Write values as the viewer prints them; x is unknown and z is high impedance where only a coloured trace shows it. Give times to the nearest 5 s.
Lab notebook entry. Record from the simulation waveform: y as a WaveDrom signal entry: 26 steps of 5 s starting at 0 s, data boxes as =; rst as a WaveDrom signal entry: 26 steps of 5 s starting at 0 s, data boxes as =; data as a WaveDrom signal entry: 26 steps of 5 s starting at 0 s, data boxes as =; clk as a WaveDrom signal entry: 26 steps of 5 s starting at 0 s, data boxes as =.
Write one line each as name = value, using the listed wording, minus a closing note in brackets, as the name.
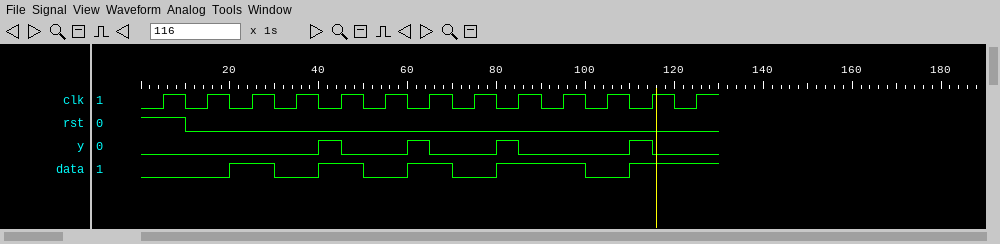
y as a WaveDrom signal entry: 26 steps of 5 s starting at 0 s, data boxes as = = {name: 'y', wave: '0.......10..10..10....10..'}
rst as a WaveDrom signal entry: 26 steps of 5 s starting at 0 s, data boxes as = = {name: 'rst', wave: '1.0.......................'}
data as a WaveDrom signal entry: 26 steps of 5 s starting at 0 s, data boxes as = = {name: 'data', wave: '0...1.0.1.0.1.0.1...0.1...'}
clk as a WaveDrom signal entry: 26 steps of 5 s starting at 0 s, data boxes as = = {name: 'clk', wave: '01010101010101010101010101'}
